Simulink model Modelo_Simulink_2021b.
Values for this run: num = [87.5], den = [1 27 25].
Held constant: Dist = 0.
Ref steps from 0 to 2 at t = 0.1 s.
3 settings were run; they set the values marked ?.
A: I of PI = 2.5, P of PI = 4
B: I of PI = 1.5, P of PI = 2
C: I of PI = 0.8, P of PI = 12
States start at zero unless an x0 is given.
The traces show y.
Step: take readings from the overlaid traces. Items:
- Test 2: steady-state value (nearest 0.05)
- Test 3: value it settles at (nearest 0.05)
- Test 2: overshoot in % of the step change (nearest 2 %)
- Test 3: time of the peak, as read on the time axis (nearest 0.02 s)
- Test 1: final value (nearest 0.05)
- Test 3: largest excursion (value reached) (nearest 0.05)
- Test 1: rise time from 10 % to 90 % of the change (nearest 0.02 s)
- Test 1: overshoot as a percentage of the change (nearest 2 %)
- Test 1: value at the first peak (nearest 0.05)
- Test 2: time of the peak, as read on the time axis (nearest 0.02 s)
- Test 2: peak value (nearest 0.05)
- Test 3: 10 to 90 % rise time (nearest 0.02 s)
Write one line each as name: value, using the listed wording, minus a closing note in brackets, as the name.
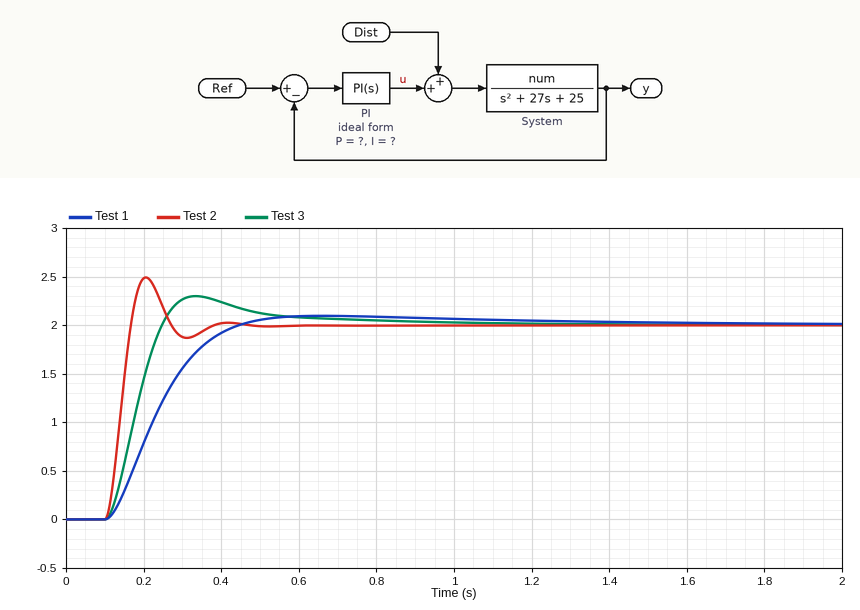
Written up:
Test 2: steady-state value: 2.00
Test 3: value it settles at: 2.00
Test 2: overshoot in % of the step change: 24 %
Test 3: time of the peak, as read on the time axis: 0.34 s
Test 1: final value: 2.00
Test 3: largest excursion (value reached): 2.30
Test 1: rise time from 10 % to 90 % of the change: 0.22 s
Test 1: overshoot as a percentage of the change: 4 %
Test 1: value at the first peak: 2.10
Test 2: time of the peak, as read on the time axis: 0.20 s
Test 2: peak value: 2.50
Test 3: 10 to 90 % rise time: 0.10 s
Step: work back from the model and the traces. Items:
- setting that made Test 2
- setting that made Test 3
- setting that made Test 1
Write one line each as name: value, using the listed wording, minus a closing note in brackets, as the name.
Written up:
setting that made Test 2: C
setting that made Test 3: A
setting that made Test 1: B
